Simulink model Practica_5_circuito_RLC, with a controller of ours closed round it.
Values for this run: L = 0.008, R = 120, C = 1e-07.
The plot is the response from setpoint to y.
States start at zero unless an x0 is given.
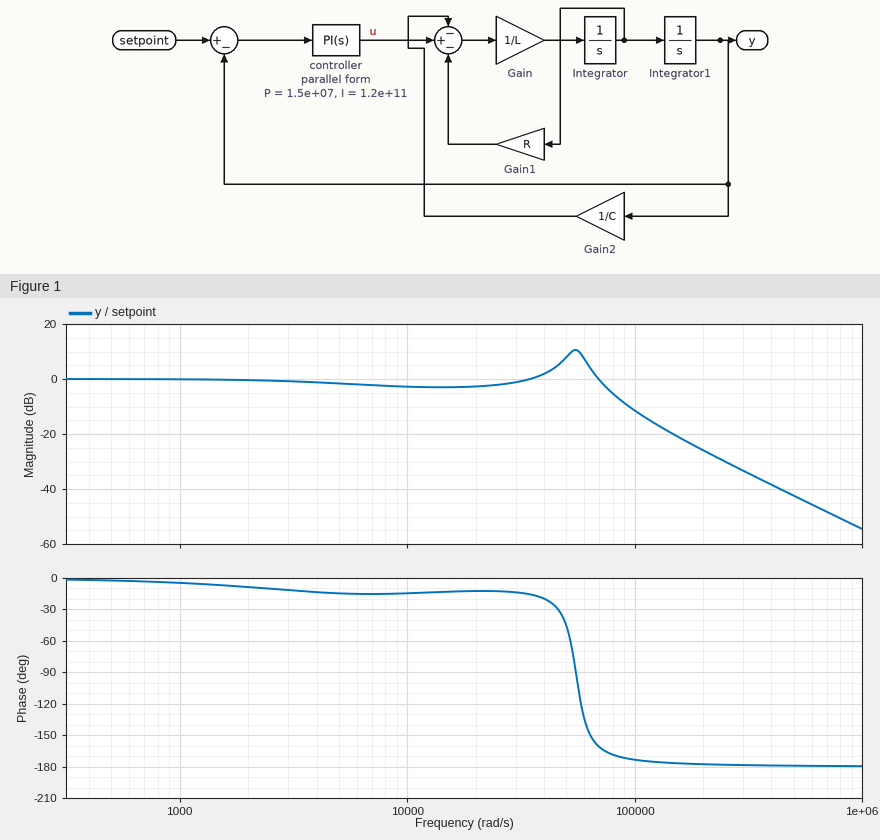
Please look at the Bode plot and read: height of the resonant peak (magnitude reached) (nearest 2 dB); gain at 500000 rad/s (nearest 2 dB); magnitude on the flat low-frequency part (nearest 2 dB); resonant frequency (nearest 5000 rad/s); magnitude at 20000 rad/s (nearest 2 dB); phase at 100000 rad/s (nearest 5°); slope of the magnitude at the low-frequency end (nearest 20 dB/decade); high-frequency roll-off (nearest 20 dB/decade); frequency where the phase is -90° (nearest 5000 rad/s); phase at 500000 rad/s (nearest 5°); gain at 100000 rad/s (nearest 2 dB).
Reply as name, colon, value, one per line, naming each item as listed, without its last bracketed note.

height of the resonant peak (magnitude reached): 10 dB
gain at 500000 rad/s: -42 dB
magnitude on the flat low-frequency part: 0 dB
resonant frequency: 55000 rad/s
magnitude at 20000 rad/s: -2 dB
phase at 100000 rad/s: -175°
slope of the magnitude at the low-frequency end: 0 dB/decade
high-frequency roll-off: -40 dB/decade
frequency where the phase is -90°: 55000 rad/s
phase at 500000 rad/s: -180°
gain at 100000 rad/s: -12 dB
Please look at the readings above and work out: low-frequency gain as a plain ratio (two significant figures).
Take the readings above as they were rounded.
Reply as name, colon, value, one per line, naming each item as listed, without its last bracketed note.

low-frequency gain as a plain ratio: 1.0
